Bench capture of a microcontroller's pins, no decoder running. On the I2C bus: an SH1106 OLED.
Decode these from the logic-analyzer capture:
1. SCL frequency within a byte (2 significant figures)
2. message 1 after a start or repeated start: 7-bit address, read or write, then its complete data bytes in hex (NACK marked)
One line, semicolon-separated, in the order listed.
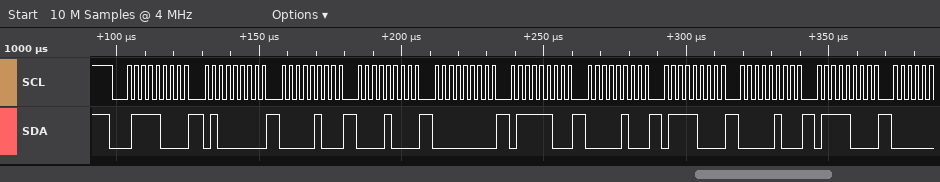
400 kHz; 0x3C write: 40 04 08 00 7C 04 78 04 78
